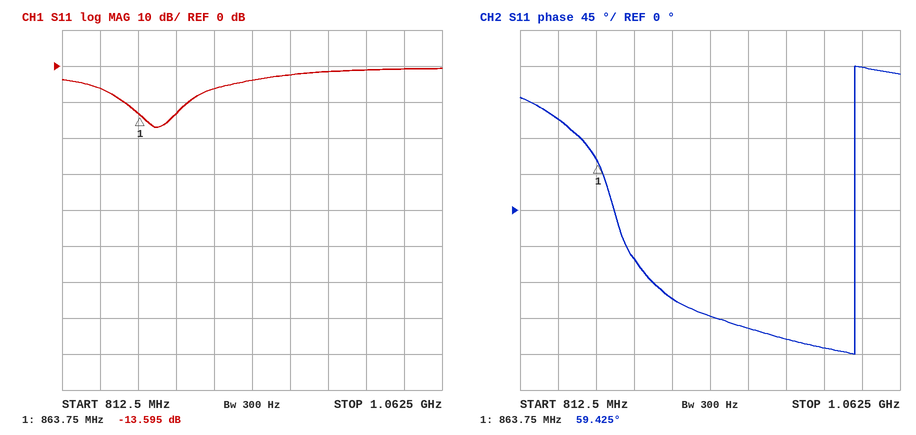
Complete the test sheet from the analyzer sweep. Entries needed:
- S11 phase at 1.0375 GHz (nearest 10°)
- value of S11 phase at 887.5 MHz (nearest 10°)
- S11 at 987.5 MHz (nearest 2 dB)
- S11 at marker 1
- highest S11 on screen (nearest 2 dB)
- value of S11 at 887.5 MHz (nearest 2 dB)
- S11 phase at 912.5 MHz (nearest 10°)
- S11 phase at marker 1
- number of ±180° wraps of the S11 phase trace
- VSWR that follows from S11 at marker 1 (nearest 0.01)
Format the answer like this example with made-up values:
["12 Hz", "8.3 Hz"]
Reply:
["180°", "-60°", "-2 dB", "-13.595 dB", "0 dB", "-14 dB", "-110°", "59.425°", "1", "1.53"]
